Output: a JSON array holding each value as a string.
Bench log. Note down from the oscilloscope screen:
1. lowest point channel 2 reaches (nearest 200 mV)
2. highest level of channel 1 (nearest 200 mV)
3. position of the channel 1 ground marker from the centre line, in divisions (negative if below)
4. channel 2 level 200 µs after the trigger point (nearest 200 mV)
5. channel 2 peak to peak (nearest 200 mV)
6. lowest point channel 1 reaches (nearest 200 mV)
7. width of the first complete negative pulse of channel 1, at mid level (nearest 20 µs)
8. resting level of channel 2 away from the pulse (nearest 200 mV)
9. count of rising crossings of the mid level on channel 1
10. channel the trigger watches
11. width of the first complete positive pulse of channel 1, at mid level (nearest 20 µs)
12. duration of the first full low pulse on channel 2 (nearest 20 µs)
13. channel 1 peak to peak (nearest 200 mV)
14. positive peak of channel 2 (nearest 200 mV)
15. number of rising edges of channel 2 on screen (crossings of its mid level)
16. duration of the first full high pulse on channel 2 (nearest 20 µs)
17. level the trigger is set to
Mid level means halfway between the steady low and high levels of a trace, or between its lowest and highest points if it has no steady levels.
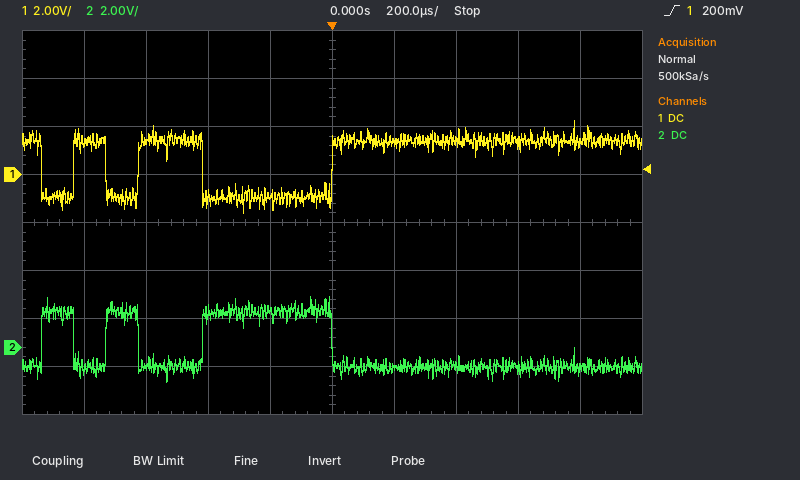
["-1.4 V", "2.2 V", "+1.0 div", "-800 mV", "3.6 V", "-1.6 V", "100 µs", "-800 mV", "3", "channel 1", "100 µs", "100 µs", "3.8 V", "2.2 V", "3", "100 µs", "200 mV"]
